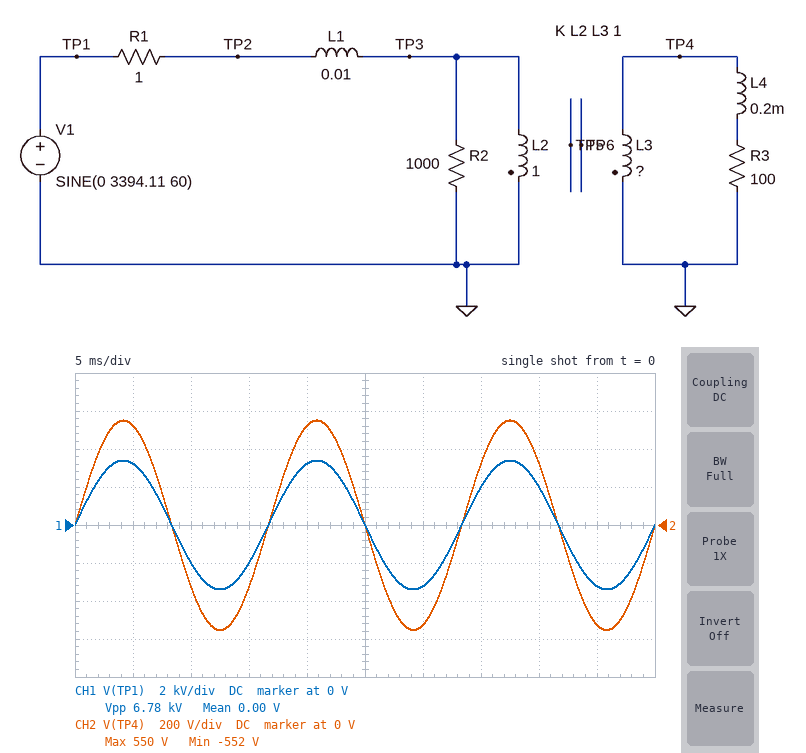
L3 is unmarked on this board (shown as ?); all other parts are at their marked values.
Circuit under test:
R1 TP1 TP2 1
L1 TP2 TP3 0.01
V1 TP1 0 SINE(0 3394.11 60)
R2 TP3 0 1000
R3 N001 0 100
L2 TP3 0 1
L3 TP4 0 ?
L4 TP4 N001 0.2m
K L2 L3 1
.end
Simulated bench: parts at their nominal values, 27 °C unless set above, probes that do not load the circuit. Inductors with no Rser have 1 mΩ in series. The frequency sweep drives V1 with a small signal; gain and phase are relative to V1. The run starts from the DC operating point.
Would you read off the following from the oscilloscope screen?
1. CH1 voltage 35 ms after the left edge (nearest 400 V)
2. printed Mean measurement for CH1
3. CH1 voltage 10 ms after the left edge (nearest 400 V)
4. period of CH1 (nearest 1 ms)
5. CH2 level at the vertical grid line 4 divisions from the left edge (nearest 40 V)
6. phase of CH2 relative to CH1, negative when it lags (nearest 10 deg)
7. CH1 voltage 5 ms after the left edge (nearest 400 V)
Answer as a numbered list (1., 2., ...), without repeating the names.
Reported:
1. 2.0 kV
2. 0.00 V
3. -2.0 kV
4. 17 ms
5. 520 V
6. 0 deg
7. 3.2 kV
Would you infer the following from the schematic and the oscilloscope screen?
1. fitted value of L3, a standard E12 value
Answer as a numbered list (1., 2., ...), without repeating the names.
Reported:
1. 27 mH
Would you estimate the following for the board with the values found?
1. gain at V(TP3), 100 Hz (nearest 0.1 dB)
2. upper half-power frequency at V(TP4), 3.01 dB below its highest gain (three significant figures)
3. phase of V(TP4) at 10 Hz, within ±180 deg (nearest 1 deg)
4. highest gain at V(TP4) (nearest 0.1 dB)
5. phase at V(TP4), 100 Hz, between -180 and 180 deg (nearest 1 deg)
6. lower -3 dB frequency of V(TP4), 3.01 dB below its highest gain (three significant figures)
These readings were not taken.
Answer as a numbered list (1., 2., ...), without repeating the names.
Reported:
1. -0.1 dB
2. 12.3 kHz
3. 1 deg
4. -15.8 dB
5. 0 deg
6. 158 mHz
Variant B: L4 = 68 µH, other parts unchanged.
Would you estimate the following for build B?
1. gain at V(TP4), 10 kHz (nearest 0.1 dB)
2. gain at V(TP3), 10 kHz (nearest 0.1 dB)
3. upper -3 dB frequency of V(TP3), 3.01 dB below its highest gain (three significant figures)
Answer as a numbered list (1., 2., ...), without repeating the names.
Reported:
1. -17.9 dB
2. -2.2 dB
3. 12.5 kHz
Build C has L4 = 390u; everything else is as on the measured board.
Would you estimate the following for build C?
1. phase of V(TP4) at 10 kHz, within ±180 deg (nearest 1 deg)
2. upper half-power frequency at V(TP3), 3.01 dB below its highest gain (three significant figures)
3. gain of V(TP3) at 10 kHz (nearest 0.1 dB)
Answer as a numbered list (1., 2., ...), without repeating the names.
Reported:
1. -37 deg
2. 12.1 kHz
3. -2.4 dB
